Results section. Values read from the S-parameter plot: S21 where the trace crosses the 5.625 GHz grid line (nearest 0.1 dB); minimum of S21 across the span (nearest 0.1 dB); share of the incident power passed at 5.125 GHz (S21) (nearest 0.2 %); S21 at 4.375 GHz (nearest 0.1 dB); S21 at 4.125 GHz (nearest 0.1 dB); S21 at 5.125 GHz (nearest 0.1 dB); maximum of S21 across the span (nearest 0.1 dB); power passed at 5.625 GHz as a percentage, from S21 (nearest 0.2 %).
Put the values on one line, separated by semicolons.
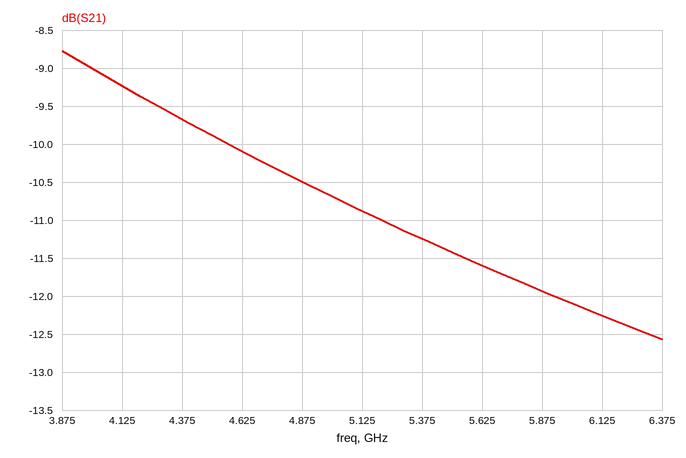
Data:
-11.6 dB; -12.6 dB; 8.2 %; -9.7 dB; -9.2 dB; -10.9 dB; -8.8 dB; 7.0 %
